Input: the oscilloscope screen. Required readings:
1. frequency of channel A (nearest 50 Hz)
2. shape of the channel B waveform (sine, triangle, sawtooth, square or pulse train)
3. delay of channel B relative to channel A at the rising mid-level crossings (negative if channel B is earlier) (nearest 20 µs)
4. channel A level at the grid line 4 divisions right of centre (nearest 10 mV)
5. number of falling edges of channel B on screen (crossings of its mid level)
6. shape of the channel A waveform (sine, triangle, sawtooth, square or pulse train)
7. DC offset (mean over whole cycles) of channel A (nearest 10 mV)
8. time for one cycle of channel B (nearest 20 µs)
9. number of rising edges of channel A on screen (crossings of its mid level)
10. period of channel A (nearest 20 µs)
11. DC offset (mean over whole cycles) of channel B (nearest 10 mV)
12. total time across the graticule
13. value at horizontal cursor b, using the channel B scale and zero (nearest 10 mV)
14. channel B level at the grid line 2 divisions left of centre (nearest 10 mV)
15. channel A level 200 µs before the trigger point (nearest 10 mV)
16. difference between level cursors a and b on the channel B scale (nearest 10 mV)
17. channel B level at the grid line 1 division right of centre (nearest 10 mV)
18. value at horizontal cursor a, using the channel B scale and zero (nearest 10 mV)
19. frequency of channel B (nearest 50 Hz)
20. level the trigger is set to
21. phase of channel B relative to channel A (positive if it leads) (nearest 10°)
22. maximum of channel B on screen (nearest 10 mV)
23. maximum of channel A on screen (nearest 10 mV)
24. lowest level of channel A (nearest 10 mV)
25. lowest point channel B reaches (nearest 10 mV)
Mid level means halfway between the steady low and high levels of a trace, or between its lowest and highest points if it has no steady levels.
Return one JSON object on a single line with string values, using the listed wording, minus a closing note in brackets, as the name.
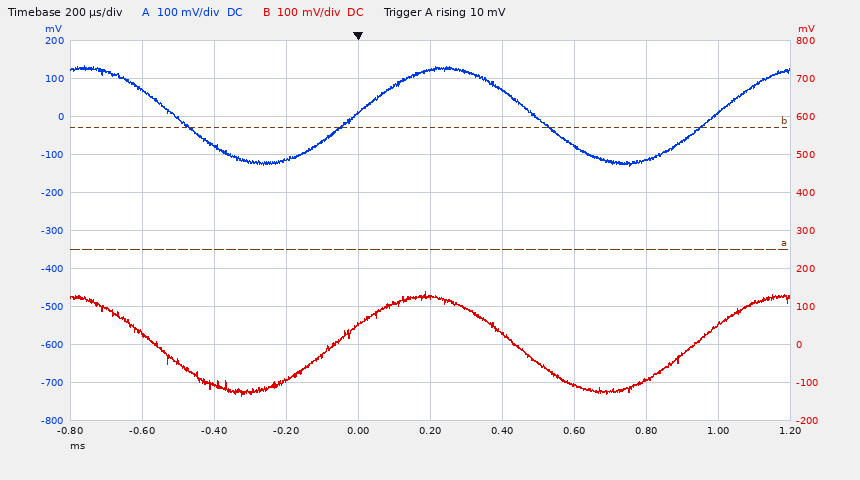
{"frequency of channel A": "1.00 kHz", "shape of the channel B waveform": "sine", "delay of channel B relative to channel A at the rising mid-level crossings (negative if channel B is earlier)": "-60 µs", "channel A level at the grid line 4 divisions right of centre": "10 mV", "number of falling edges of channel B on screen": "2", "shape of the channel A waveform": "sine", "DC offset (mean over whole cycles) of channel A": "0 mV", "time for one cycle of channel B": "1.00 ms", "number of rising edges of channel A on screen": "2", "period of channel A": "1.00 ms", "DC offset (mean over whole cycles) of channel B": "0 mV", "total time across the graticule": "2 ms", "value at horizontal cursor b, using the channel B scale and zero": "570 mV", "channel B level at the grid line 2 divisions left of centre": "-90 mV", "channel A level 200 µs before the trigger point": "-120 mV", "difference between level cursors a and b on the channel B scale": "320 mV", "channel B level at the grid line 1 division right of centre": "30 mV", "value at horizontal cursor a, using the channel B scale and zero": "250 mV", "frequency of channel B": "1.00 kHz", "level the trigger is set to": "10 mV", "phase of channel B relative to channel A (positive if it leads)": "+20°", "maximum of channel B on screen": "140 mV", "maximum of channel A on screen": "130 mV", "lowest level of channel A": "-130 mV", "lowest point channel B reaches": "-140 mV"}
